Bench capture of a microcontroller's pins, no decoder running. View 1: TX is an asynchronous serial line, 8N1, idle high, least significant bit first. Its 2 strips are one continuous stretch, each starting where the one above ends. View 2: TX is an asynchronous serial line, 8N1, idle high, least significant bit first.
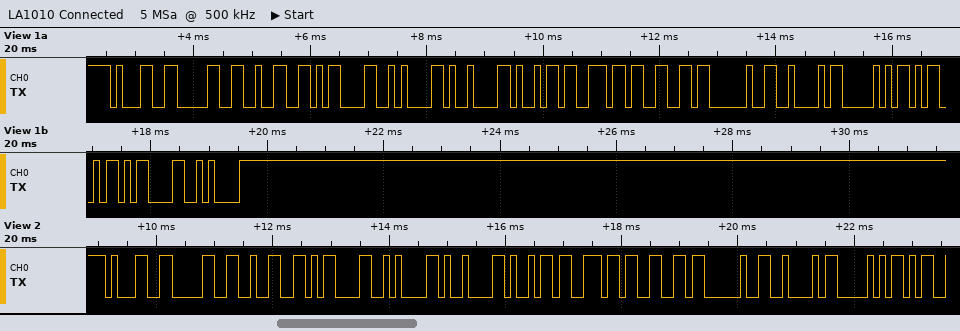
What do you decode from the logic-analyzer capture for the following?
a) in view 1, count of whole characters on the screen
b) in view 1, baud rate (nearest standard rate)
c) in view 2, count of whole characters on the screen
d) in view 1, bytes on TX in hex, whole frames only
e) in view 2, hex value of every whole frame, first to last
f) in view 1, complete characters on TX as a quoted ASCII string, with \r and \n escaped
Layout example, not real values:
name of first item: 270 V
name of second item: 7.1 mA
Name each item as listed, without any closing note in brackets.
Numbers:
in view 1, count of whole characters on the screen: 15
in view 1, baud rate: 9600 baud
in view 2, count of whole characters on the screen: 12
in view 1, bytes on TX in hex, whole frames only: 31 30 32 0D 0A 09 69 6E 66 20 42 50 4D 0D 0A
in view 2, hex value of every whole frame, first to last: 31 30 32 0D 0A 09 69 6E 66 20 42 50
in view 1, complete characters on TX as a quoted ASCII string, with \r and \n escaped: "102\r\n\tinf BPM\r\n"
